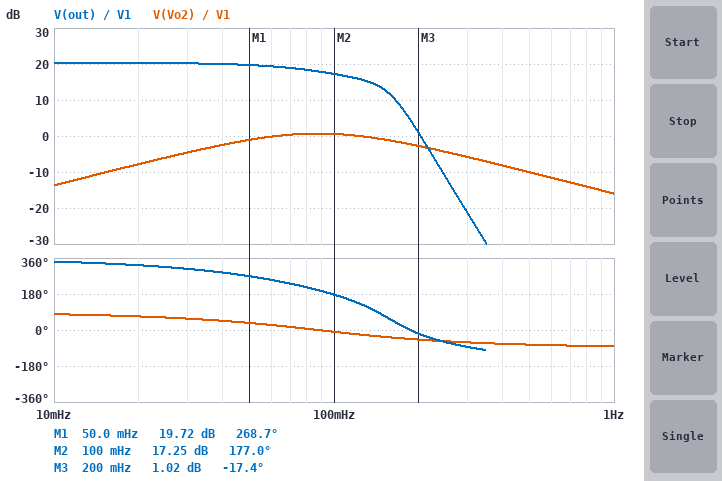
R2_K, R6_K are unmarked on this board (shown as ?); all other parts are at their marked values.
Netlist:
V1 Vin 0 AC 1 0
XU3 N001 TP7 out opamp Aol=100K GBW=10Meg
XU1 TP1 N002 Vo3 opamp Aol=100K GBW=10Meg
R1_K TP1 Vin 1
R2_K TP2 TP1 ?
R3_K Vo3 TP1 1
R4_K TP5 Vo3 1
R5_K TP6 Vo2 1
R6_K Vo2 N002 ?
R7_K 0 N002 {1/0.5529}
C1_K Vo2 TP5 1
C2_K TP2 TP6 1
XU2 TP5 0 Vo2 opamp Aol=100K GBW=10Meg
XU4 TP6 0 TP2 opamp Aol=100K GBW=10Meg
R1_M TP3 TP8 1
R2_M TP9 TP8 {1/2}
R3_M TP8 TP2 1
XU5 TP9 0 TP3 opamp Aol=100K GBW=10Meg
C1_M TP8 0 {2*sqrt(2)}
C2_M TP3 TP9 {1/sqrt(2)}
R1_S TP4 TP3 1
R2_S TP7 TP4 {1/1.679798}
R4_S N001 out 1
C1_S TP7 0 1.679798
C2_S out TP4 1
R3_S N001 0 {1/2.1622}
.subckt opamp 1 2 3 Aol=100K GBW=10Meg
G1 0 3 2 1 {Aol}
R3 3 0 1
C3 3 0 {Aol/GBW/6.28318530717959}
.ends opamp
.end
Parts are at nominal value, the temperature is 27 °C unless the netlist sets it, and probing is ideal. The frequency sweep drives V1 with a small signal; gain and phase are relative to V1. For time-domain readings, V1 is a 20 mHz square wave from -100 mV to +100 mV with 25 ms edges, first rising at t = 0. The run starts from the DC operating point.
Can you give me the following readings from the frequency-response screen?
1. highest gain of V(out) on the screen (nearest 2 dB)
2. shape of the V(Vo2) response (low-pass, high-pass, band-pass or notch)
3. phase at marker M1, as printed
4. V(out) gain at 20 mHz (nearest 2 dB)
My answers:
20 dB
band-pass
268.7 deg
20 dB
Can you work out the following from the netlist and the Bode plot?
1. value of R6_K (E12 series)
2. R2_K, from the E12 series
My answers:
2.7 Ω
3.3 Ω
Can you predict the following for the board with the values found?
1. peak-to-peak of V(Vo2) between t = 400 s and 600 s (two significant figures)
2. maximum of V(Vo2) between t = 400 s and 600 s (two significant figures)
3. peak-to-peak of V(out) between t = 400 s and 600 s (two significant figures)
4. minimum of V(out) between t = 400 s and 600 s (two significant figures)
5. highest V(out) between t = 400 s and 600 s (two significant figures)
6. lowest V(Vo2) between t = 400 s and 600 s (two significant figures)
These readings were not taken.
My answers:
300 mV
150 mV
2.2 V
-1.1 V
1.1 V
-150 mV
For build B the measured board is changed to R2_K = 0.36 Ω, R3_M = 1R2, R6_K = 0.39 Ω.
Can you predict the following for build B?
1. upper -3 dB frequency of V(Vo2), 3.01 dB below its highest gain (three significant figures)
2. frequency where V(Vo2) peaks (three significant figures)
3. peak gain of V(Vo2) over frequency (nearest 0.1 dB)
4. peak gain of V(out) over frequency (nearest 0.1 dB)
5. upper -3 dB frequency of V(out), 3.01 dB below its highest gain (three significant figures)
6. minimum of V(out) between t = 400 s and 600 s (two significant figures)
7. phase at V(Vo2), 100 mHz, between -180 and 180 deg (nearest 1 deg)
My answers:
723 mHz
265 mHz
-11.9 dB
0.9 dB
165 mHz
-130 mV
44 deg
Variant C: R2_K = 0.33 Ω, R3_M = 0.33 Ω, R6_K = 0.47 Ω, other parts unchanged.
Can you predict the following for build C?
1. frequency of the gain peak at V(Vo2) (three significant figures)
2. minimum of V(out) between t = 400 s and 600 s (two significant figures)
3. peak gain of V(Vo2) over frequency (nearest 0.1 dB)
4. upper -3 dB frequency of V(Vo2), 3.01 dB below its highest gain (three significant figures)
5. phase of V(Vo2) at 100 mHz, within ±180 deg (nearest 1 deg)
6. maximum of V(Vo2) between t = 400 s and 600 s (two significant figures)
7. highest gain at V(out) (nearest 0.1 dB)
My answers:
277 mHz
-340 mV
-12.0 dB
739 mHz
46 deg
39 mV
10.0 dB
